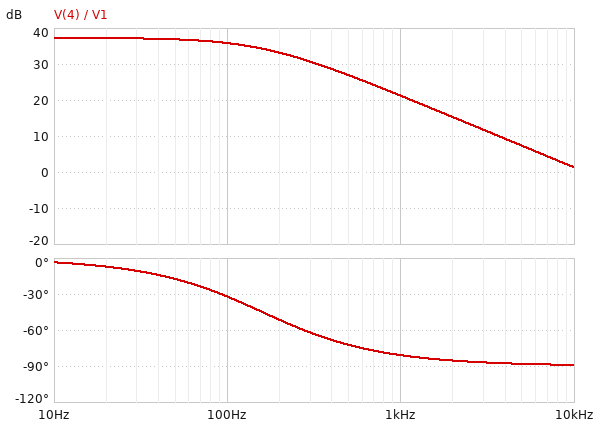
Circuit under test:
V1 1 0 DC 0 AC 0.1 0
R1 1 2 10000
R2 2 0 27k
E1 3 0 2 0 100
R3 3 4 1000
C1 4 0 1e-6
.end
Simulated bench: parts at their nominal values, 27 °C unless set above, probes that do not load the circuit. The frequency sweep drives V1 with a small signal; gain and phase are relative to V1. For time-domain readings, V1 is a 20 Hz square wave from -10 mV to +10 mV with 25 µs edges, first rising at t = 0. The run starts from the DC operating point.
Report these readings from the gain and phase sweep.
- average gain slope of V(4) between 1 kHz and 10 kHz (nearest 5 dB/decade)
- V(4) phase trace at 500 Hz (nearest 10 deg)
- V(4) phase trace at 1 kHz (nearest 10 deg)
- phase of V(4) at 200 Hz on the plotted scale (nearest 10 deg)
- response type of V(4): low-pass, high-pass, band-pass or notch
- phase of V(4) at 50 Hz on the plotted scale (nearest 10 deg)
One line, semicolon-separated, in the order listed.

-20 dB/decade; -70 deg; -80 deg; -50 deg; low-pass; -20 deg
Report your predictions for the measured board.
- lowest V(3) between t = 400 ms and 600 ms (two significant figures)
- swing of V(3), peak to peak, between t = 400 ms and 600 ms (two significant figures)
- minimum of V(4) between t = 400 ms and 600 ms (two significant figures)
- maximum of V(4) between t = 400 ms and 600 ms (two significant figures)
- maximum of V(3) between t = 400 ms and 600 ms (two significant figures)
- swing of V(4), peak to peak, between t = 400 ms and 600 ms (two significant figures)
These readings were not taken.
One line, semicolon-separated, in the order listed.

-730 mV; 1.5 V; -730 mV; 730 mV; 730 mV; 1.5 V
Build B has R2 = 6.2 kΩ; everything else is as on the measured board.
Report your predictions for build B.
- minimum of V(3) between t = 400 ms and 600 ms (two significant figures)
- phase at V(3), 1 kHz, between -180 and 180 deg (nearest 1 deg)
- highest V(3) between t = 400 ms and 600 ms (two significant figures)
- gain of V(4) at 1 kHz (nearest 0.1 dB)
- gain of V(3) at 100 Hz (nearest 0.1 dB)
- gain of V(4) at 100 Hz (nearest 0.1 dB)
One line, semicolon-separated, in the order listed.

-380 mV; 0 deg; 380 mV; 15.6 dB; 31.7 dB; 30.2 dB
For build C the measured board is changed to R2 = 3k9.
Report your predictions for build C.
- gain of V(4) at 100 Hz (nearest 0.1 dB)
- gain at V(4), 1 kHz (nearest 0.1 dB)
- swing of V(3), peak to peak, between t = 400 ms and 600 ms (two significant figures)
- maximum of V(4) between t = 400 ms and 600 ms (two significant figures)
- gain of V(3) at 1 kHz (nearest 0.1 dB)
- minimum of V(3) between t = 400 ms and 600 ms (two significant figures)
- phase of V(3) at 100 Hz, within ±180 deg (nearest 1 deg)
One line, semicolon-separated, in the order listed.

27.5 dB; 12.9 dB; 560 mV; 280 mV; 29.0 dB; -280 mV; 0 deg
